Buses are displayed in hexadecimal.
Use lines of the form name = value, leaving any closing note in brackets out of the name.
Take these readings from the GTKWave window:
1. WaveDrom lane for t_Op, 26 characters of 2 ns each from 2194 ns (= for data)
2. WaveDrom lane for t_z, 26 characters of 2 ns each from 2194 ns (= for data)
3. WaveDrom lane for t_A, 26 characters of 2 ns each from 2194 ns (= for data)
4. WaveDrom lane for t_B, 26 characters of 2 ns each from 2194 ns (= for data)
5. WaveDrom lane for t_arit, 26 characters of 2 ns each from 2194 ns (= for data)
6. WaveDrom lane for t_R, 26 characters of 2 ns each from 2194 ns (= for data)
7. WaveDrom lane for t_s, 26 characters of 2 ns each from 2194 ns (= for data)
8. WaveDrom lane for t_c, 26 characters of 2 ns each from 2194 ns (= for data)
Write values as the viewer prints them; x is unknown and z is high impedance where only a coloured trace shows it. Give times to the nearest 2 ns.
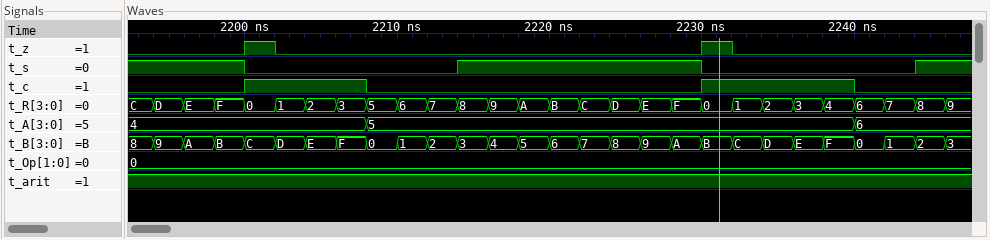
WaveDrom lane for t_Op, 26 characters of 2 ns each from 2194 ns = {name: 't_Op', wave: '=.........................', data: '0'}
WaveDrom lane for t_z, 26 characters of 2 ns each from 2194 ns = {name: 't_z', wave: '0..10.............10......'}
WaveDrom lane for t_A, 26 characters of 2 ns each from 2194 ns = {name: 't_A', wave: '=......=...............=..', data: '4 5 6'}
WaveDrom lane for t_B, 26 characters of 2 ns each from 2194 ns = {name: 't_B', wave: '==========================', data: '9 A B C D E F 0 1 2 3 4 5 6 7 8 9 A B C D E F 0 1 2'}
WaveDrom lane for t_arit, 26 characters of 2 ns each from 2194 ns = {name: 't_arit', wave: '1.........................'}
WaveDrom lane for t_R, 26 characters of 2 ns each from 2194 ns = {name: 't_R', wave: '==========================', data: 'D E F 0 1 2 3 5 6 7 8 9 A B C D E F 0 1 2 3 4 6 7 8'}
WaveDrom lane for t_s, 26 characters of 2 ns each from 2194 ns = {name: 't_s', wave: '1..0......1.......0......1'}
WaveDrom lane for t_c, 26 characters of 2 ns each from 2194 ns = {name: 't_c', wave: '0..1...0..........1....0..'}
